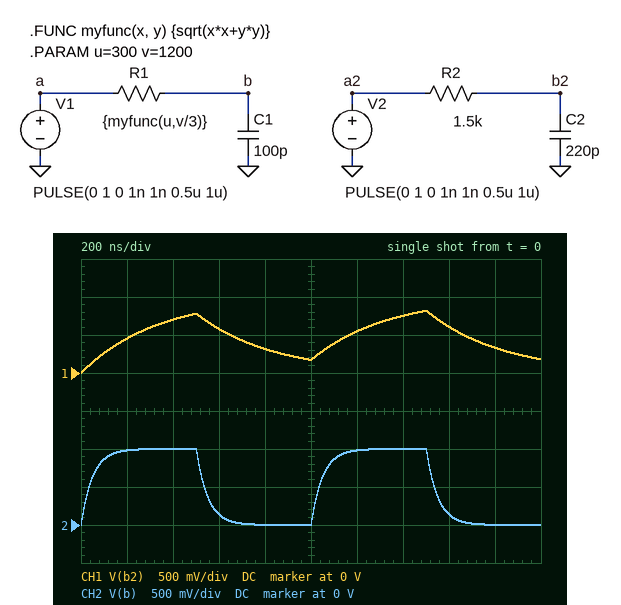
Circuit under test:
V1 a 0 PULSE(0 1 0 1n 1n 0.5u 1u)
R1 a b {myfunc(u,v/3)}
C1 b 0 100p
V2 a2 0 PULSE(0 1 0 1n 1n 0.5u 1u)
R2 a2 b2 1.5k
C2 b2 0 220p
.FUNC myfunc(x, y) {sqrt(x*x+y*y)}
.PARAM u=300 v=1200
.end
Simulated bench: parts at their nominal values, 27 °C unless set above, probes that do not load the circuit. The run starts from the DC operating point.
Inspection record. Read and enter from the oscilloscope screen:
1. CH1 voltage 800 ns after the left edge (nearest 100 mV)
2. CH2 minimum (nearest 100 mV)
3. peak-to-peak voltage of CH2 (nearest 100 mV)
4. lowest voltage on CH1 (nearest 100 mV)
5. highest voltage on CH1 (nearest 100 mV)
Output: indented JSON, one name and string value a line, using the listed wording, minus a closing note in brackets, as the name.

{
  "CH1 voltage 800 ns after the left edge": "300 mV",
  "CH2 minimum": "0 V",
  "peak-to-peak voltage of CH2": "1.0 V",
  "lowest voltage on CH1": "0 V",
  "highest voltage on CH1": "800 mV"
}
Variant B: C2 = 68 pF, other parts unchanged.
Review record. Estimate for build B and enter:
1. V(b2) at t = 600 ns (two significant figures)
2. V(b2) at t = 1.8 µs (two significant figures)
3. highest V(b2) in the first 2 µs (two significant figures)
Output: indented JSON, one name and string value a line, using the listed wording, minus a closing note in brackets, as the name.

{
  "V(b2) at t = 600 ns": "380 mV",
  "V(b2) at t = 1.8 µs": "53 mV",
  "highest V(b2) in the first 2 µs": "990 mV"
}
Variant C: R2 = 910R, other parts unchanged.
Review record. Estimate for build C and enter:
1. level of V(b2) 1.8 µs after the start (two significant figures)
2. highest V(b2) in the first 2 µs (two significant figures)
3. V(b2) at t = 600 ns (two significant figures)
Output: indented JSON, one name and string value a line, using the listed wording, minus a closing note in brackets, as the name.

{
  "level of V(b2) 1.8 µs after the start": "210 mV",
  "highest V(b2) in the first 2 µs": "920 mV",
  "V(b2) at t = 600 ns": "560 mV"
}
